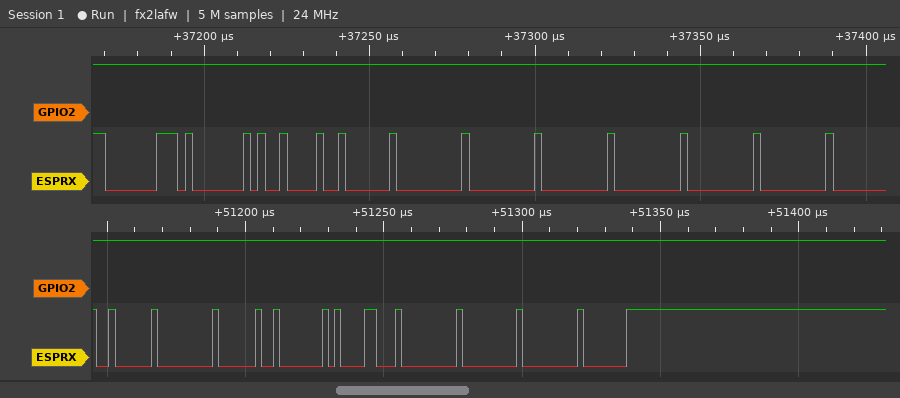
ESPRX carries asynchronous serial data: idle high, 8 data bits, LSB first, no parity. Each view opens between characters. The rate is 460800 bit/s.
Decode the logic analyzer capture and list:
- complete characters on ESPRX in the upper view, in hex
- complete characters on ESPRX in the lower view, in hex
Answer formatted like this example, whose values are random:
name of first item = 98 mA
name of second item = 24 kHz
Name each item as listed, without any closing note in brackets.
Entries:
complete characters on ESPRX in the upper view, in hex = C0, 01, 09, 02, 00, 00, 00, 00, 00, 00
complete characters on ESPRX in the lower view, in hex = 02, 00, 20, 40, 18, 00, 00, 00, C0
